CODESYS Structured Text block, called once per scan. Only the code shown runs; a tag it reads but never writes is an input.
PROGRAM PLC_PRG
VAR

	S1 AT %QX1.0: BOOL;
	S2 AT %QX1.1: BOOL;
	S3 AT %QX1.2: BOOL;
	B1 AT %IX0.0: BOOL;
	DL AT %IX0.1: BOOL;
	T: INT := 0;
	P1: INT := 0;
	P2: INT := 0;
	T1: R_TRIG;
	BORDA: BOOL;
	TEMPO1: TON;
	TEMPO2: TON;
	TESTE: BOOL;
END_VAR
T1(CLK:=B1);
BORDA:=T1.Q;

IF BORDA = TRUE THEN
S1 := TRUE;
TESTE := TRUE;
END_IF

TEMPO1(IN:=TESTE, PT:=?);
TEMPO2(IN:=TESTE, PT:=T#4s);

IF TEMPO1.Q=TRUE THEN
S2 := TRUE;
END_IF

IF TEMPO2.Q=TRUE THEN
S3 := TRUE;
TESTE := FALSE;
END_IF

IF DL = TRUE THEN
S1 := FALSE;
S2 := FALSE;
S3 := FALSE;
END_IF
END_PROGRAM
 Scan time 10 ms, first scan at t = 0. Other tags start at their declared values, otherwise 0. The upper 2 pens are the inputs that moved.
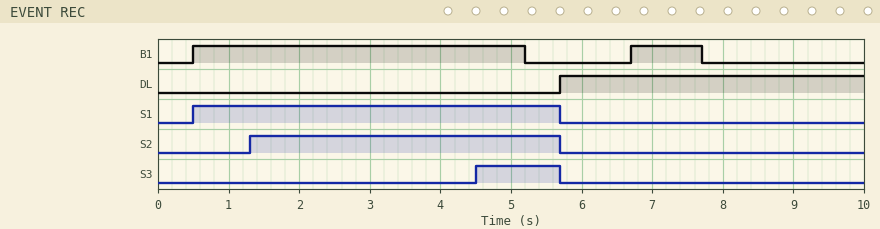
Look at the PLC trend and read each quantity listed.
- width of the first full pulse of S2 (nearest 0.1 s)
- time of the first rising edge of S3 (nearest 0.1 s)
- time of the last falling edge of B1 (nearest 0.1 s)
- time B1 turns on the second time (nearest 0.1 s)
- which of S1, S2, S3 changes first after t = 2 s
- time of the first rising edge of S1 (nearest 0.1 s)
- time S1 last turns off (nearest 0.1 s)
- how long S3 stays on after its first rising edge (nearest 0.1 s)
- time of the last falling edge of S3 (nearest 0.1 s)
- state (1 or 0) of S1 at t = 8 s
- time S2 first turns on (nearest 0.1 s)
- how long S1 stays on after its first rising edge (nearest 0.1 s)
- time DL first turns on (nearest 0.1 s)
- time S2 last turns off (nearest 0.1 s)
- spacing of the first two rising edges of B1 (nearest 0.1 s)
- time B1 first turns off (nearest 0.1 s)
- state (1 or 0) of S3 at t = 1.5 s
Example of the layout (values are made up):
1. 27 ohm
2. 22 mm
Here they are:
1. 4.4 s
2. 4.5 s
3. 7.7 s
4. 6.7 s
5. S3
6. 0.5 s
7. 5.7 s
8. 1.2 s
9. 5.7 s
10. 0
11. 1.3 s
12. 5.2 s
13. 5.7 s
14. 5.7 s
15. 6.2 s
16. 5.2 s
17. 0
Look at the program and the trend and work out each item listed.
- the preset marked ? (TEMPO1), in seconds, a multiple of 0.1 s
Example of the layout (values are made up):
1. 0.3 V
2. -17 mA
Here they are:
1. 0.8 s
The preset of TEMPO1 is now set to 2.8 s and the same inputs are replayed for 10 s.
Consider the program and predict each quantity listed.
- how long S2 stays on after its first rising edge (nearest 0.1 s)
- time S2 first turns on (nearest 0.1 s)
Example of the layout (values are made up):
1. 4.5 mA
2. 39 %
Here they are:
1. 2.4 s
2. 3.3 s
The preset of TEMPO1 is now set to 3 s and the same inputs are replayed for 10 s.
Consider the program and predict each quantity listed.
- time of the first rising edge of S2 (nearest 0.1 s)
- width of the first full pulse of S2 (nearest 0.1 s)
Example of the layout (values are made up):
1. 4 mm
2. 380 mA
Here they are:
1. 3.5 s
2. 2.2 s
